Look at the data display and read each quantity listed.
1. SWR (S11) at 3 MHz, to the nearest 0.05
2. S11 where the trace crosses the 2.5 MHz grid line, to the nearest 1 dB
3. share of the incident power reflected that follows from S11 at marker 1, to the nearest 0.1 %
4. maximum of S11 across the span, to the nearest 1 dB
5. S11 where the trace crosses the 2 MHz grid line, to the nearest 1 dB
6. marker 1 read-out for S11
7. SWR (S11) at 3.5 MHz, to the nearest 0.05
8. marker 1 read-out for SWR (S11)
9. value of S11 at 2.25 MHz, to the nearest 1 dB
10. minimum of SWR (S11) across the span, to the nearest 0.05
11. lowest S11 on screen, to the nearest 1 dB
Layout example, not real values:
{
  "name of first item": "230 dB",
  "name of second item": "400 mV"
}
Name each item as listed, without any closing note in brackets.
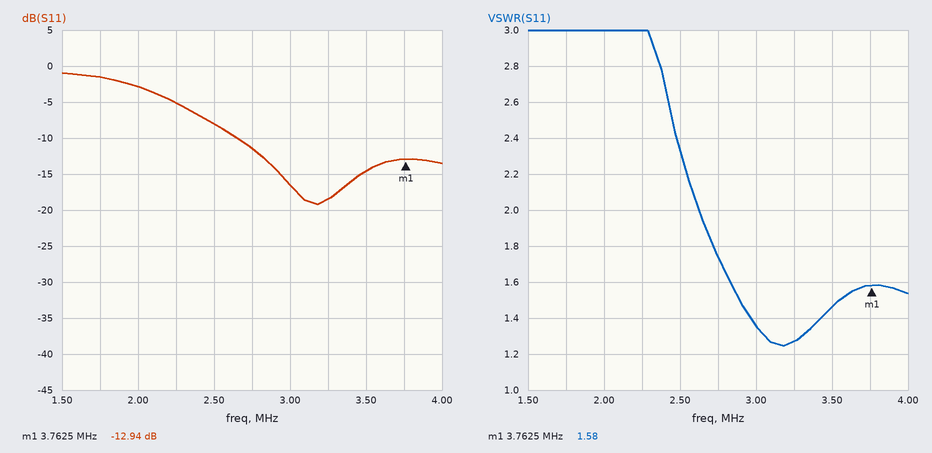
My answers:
{
  "SWR (S11) at 3 MHz, to the nearest 0.05": "1.35",
  "S11 where the trace crosses the 2.5 MHz grid line, to the nearest 1 dB": "-8 dB",
  "share of the incident power reflected that follows from S11 at marker 1, to the nearest 0.1 %": "5.1 %",
  "maximum of S11 across the span, to the nearest 1 dB": "-1 dB",
  "S11 where the trace crosses the 2 MHz grid line, to the nearest 1 dB": "-3 dB",
  "marker 1 read-out for S11": "-12.94 dB",
  "SWR (S11) at 3.5 MHz, to the nearest 0.05": "1.45",
  "marker 1 read-out for SWR": "1.58",
  "value of S11 at 2.25 MHz, to the nearest 1 dB": "-5 dB",
  "minimum of SWR (S11) across the span, to the nearest 0.05": "1.25",
  "lowest S11 on screen, to the nearest 1 dB": "-19 dB"
}
